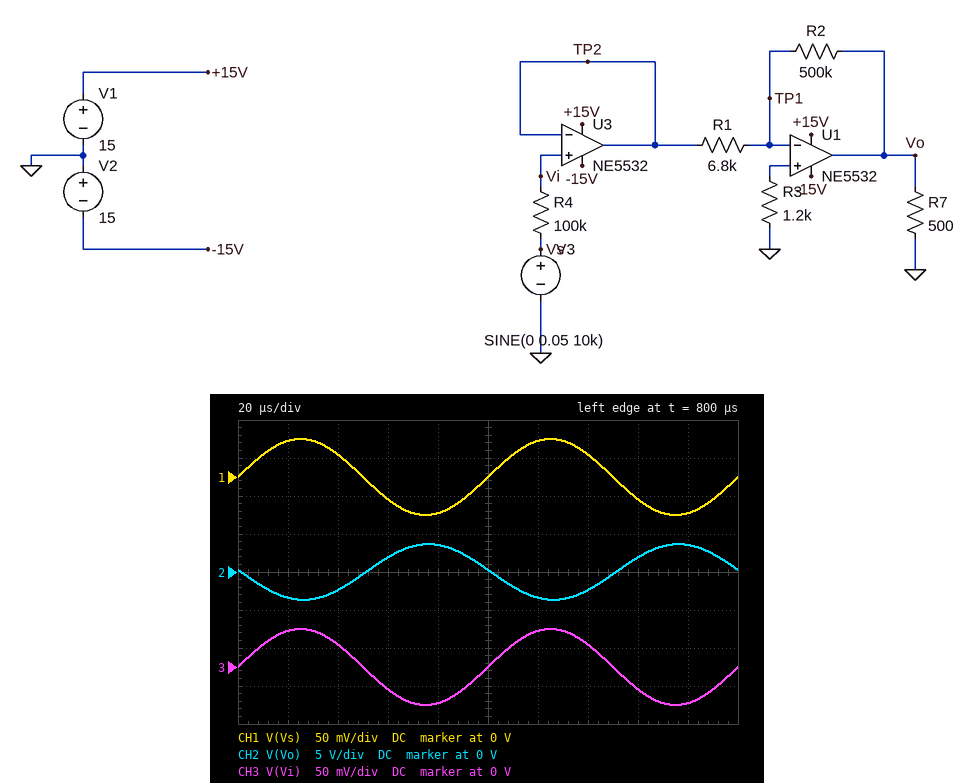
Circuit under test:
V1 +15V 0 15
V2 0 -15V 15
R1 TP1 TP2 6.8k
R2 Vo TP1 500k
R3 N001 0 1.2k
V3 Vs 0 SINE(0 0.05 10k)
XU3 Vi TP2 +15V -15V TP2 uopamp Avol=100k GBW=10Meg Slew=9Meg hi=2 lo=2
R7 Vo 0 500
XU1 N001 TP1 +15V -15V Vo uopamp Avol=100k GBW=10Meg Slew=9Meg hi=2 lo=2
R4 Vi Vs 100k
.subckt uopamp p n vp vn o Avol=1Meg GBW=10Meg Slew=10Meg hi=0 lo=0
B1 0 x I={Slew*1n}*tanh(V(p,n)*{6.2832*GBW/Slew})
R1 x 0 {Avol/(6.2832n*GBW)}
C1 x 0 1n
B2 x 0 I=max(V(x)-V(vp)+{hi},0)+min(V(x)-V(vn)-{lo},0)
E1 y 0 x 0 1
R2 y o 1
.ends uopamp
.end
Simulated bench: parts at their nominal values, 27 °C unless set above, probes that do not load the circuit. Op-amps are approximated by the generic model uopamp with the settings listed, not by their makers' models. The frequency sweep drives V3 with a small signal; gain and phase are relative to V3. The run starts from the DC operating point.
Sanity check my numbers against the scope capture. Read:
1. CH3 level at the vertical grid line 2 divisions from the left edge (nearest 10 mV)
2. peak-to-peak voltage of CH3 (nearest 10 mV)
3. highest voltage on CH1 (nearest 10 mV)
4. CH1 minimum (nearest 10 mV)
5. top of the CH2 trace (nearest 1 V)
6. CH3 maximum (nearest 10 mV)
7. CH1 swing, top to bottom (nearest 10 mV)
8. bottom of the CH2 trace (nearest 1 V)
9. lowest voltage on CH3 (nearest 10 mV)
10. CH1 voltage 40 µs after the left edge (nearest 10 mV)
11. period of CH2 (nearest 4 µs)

30 mV
100 mV
50 mV
-50 mV
4 V
50 mV
100 mV
-4 V
-50 mV
30 mV
100 µs
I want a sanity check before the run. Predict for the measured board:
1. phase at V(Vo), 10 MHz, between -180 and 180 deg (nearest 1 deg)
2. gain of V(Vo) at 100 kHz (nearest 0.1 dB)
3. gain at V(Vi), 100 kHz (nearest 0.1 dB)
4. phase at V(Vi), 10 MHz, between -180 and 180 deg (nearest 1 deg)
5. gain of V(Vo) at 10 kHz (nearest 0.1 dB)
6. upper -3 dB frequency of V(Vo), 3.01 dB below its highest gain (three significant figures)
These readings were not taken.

46 deg
35.4 dB
0 dB
0 deg
37.3 dB
134 kHz
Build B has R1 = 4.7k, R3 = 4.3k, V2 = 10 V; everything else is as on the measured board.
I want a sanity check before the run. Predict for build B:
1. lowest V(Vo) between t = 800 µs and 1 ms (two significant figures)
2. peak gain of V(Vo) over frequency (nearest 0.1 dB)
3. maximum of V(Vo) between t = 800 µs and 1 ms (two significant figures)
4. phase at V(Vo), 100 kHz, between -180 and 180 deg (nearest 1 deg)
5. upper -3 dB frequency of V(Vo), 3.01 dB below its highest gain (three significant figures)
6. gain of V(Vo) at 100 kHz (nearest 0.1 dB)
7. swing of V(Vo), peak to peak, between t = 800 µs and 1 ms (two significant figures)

-5.3 V
40.5 dB
5.3 V
132 deg
93.0 kHz
37.2 dB
11 V
